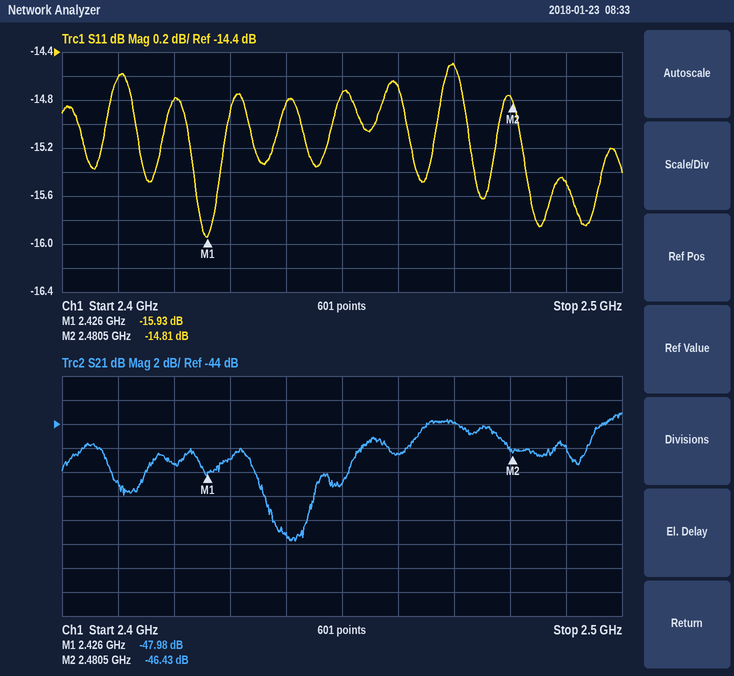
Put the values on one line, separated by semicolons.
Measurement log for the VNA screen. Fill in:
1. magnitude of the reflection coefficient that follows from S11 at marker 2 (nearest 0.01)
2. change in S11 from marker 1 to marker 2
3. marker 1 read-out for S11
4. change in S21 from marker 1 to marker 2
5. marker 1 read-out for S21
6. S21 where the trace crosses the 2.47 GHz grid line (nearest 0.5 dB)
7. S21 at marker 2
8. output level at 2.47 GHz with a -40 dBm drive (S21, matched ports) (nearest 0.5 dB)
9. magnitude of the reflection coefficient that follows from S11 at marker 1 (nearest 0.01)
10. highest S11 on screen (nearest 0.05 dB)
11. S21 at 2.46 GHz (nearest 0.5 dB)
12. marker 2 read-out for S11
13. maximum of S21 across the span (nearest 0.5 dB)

0.18; 1.12 dB; -15.93 dB; 1.55 dB; -47.98 dB; -44.0 dB; -46.43 dB; -84.0 dBm; 0.16; -14.50 dB; -46.5 dB; -14.81 dB; -43.0 dB
